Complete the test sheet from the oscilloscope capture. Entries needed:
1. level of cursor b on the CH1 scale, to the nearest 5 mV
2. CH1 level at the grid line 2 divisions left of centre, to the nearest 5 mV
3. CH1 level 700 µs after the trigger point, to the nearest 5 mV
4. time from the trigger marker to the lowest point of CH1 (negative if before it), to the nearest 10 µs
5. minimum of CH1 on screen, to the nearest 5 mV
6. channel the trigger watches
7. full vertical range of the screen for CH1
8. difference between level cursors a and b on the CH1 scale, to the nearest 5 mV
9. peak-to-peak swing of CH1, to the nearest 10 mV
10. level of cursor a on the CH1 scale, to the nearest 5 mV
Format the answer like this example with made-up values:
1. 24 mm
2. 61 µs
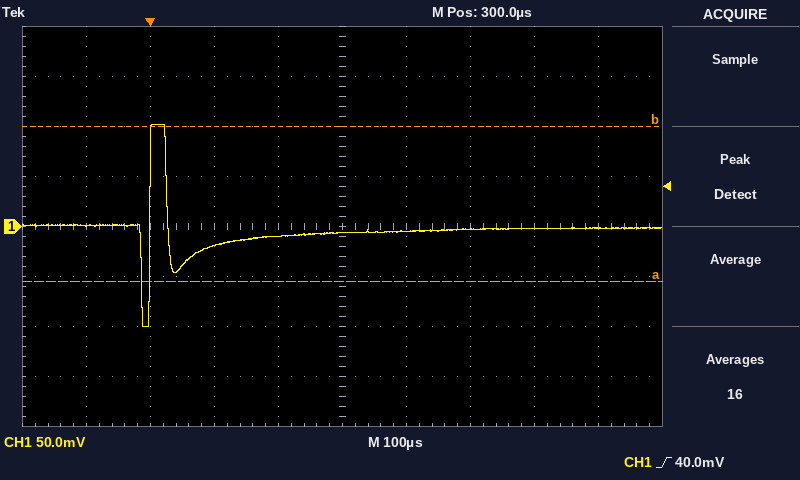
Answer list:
1. 100 mV
2. -20 mV
3. 0 mV
4. -10 µs
5. -100 mV
6. CH1
7. 400 mV
8. 155 mV
9. 200 mV
10. -55 mV
